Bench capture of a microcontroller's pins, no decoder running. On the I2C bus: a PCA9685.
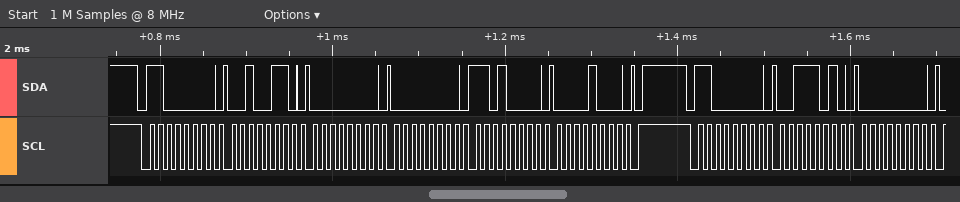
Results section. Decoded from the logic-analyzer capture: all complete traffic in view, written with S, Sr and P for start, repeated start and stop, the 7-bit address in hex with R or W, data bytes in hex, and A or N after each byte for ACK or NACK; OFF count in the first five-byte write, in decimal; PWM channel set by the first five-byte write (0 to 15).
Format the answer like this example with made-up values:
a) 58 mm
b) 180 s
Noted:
a) S 60W A 26 A 00 A 00 A D0 A 08 A P S 60W A 3A A 00 A
b) 2256
c) 8
